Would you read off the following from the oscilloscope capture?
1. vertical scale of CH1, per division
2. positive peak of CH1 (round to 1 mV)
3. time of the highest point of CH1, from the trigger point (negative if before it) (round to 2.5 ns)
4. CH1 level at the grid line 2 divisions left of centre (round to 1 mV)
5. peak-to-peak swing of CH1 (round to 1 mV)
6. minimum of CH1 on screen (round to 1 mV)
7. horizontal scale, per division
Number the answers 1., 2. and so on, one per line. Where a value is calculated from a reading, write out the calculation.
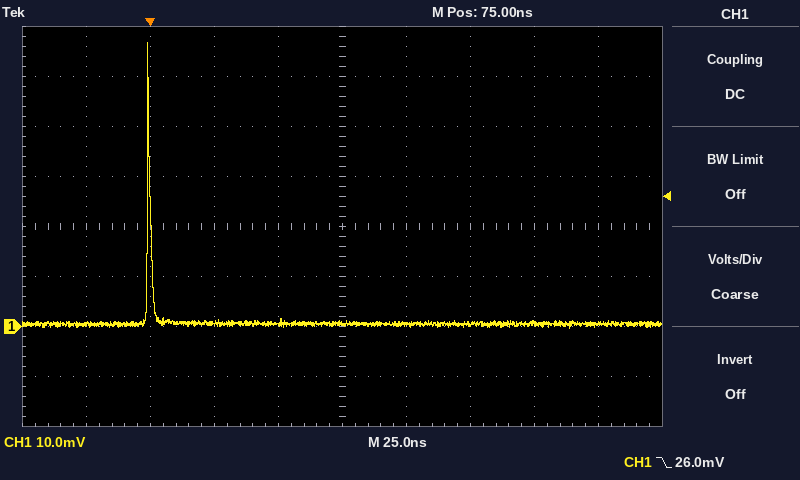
1. 10 mV
2. 57 mV
3. 0.0 ns
4. 1 mV
5. 57 mV − (0 mV) = 57 mV
6. 0 mV
7. 25 ns
